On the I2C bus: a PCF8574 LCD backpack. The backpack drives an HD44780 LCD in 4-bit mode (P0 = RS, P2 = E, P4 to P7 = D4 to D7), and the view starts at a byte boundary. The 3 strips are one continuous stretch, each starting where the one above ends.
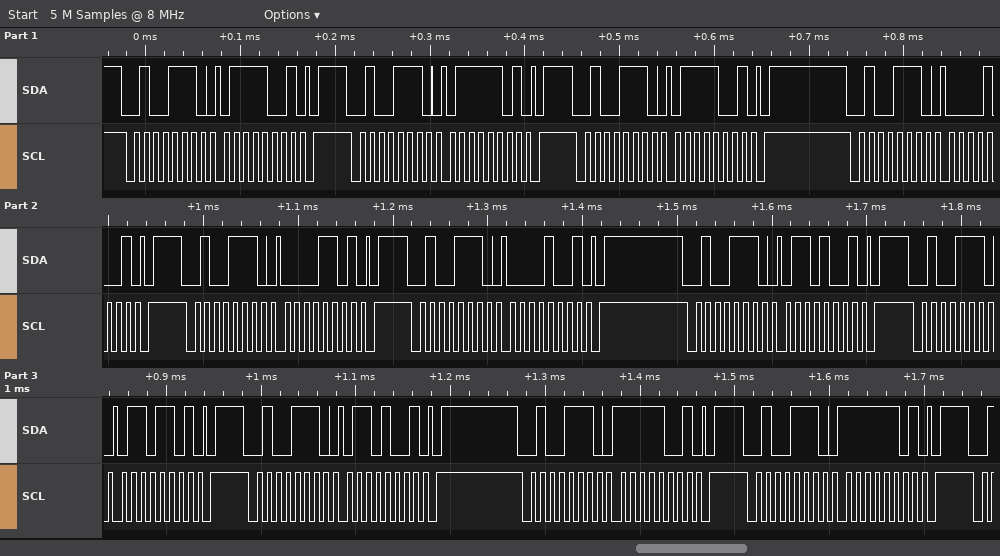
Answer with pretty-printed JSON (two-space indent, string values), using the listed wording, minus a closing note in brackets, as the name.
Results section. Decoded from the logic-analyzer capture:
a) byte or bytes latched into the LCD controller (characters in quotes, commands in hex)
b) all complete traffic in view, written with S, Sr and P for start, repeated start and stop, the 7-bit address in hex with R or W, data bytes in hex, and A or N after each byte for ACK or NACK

{
  "byte or bytes latched into the LCD controller": "'p'",
  "all complete traffic in view, written with S, Sr and P for start, repeated start and stop, the 7-bit address in hex with R or W, data bytes in hex, and A or N after each byte for ACK or NACK": "S 27W A 79 A P S 27W A 7D A P S 27W A 79 A P S 27W A 09 A P S 27W A 0D A P S 27W A 09 A P S 27W A 69 A P S 27W A 6D A P S 27W A 69 A P S 27W A F9 A P S 27W A FD A P"
}
